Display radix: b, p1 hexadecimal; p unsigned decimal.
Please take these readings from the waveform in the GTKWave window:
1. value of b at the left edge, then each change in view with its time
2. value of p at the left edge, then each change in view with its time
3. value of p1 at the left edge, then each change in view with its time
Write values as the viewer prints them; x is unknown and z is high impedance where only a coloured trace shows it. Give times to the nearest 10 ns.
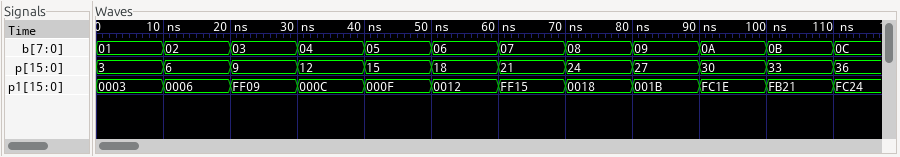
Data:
01, 02 at 10 ns, 03 at 20 ns, 04 at 30 ns, 05 at 40 ns, 06 at 50 ns, 07 at 60 ns, 08 at 70 ns, 09 at 80 ns, 0A at 90 ns, 0B at 100 ns, 0C at 110 ns
3, 6 at 10 ns, 9 at 20 ns, 12 at 30 ns, 15 at 40 ns, 18 at 50 ns, 21 at 60 ns, 24 at 70 ns, 27 at 80 ns, 30 at 90 ns, 33 at 100 ns, 36 at 110 ns
0003, 0006 at 10 ns, FF09 at 20 ns, 000C at 30 ns, 000F at 40 ns, 0012 at 50 ns, FF15 at 60 ns, 0018 at 70 ns, 001B at 80 ns, FC1E at 90 ns, FB21 at 100 ns, FC24 at 110 ns
